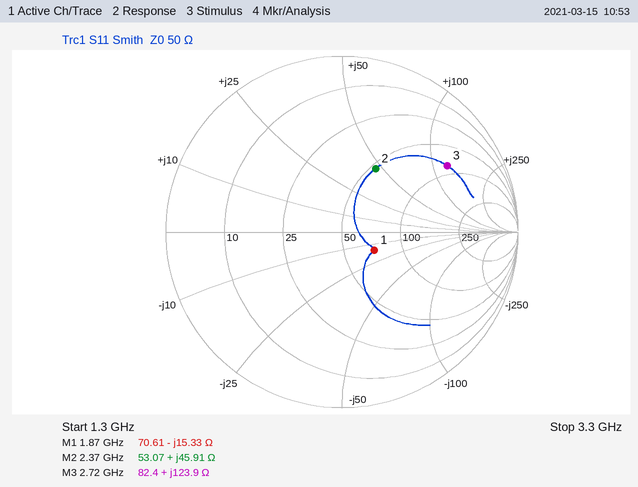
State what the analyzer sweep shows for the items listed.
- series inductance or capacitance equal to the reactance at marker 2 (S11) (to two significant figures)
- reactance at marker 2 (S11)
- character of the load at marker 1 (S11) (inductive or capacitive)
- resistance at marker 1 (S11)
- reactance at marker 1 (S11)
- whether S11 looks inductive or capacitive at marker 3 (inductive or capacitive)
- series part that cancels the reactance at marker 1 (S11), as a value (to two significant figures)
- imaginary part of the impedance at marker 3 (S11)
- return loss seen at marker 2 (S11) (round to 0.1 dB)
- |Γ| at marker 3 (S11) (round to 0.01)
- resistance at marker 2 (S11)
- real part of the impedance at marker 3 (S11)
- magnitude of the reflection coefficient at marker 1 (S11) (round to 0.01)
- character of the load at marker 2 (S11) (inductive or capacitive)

3.1 nH
+45.91 Ω
capacitive
70.61 Ω
-15.33 Ω
inductive
1.3 nH
+123.9 Ω
7.8 dB
0.71
53.07 Ω
82.4 Ω
0.21
inductive
